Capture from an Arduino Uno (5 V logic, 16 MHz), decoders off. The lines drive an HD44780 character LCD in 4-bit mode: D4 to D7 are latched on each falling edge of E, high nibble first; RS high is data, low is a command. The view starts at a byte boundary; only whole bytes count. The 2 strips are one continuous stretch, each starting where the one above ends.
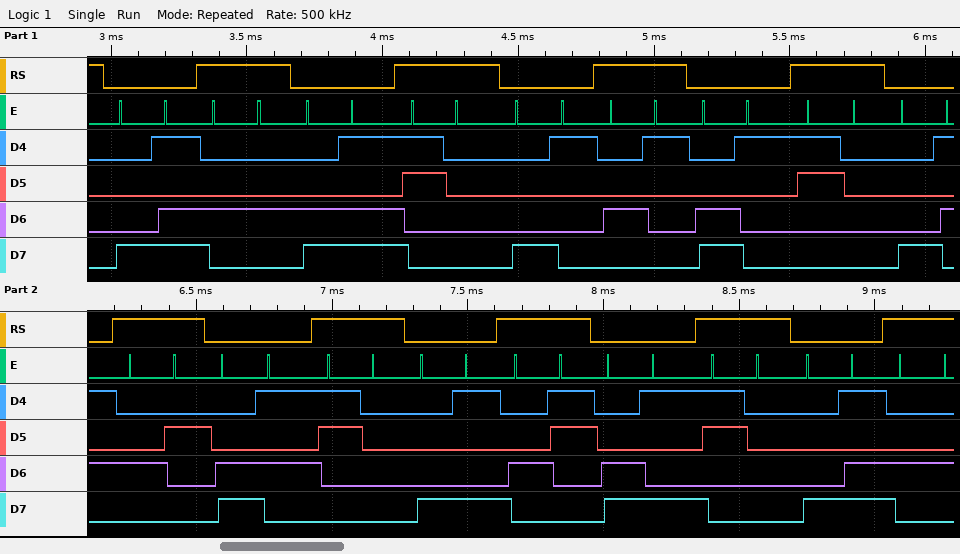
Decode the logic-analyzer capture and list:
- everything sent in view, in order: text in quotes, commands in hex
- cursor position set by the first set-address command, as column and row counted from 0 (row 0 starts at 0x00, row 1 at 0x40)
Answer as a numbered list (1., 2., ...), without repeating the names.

1. 0x8D "D" 0xCD "0" 0x81 "A" 0xC1 "0" 0x85 "B" 0xC5 "0" 0x89 "C" 0xC9 "0" 0x8D "D"
2. column 13, row 0
